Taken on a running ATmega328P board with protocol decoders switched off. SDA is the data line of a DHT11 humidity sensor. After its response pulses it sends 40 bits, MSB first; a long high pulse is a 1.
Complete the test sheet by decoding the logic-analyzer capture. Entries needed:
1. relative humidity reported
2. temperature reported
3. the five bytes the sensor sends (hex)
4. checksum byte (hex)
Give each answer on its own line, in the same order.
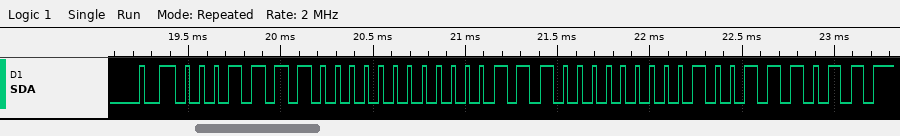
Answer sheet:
30 %
28.1 °C
1E 00 1C 01 3B
0x3B
